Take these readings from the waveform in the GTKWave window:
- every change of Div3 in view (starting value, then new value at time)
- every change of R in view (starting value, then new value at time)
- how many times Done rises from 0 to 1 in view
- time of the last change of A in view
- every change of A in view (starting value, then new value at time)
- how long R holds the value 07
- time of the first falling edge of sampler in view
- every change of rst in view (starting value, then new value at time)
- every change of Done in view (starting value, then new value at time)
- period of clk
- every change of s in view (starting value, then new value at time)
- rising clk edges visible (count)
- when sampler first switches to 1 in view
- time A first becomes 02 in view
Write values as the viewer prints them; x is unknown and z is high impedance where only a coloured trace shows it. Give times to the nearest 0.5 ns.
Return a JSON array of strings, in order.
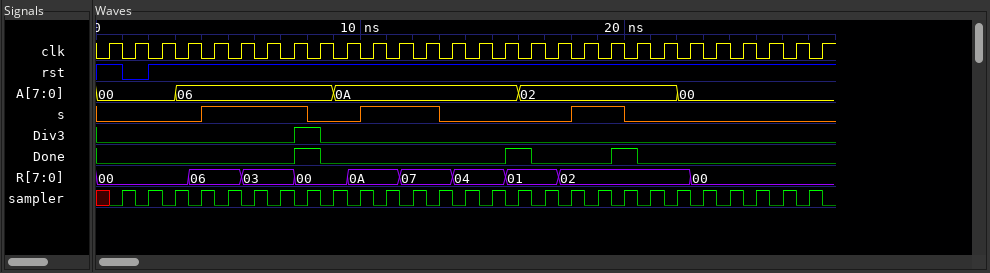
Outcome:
["0, 1 at 7.5 ns, 0 at 8.5 ns", "00, 06 at 3.5 ns, 03 at 5.5 ns, 00 at 7.5 ns, 0A at 9.5 ns, 07 at 11.5 ns, 04 at 13.5 ns, 01 at 15.5 ns, 02 at 17.5 ns, 00 at 22.5 ns", "3", "22 ns", "00, 06 at 3 ns, 0A at 9 ns, 02 at 16 ns, 00 at 22 ns", "2 ns", "1.5 ns", "1, 0 at 1 ns, 1 at 2 ns", "0, 1 at 7.5 ns, 0 at 8.5 ns, 1 at 15.5 ns, 0 at 16.5 ns, 1 at 19.5 ns, 0 at 20.5 ns", "1 ns", "0, 1 at 4 ns, 0 at 8 ns, 1 at 10 ns, 0 at 13 ns, 1 at 18 ns, 0 at 20 ns", "28", "1 ns", "16 ns"]
